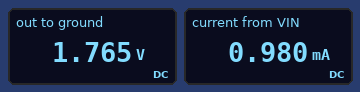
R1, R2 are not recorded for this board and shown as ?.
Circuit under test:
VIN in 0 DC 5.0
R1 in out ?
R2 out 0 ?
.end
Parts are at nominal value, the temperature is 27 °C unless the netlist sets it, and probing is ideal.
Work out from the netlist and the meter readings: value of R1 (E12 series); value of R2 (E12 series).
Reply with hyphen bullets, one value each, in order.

- 3.3 kΩ
- 1.8 kΩ
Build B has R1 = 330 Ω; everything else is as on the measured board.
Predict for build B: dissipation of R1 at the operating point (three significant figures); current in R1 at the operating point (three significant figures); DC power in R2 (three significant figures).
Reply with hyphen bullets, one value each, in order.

- 1.82 mW
- 2.35 mA
- 9.92 mW
